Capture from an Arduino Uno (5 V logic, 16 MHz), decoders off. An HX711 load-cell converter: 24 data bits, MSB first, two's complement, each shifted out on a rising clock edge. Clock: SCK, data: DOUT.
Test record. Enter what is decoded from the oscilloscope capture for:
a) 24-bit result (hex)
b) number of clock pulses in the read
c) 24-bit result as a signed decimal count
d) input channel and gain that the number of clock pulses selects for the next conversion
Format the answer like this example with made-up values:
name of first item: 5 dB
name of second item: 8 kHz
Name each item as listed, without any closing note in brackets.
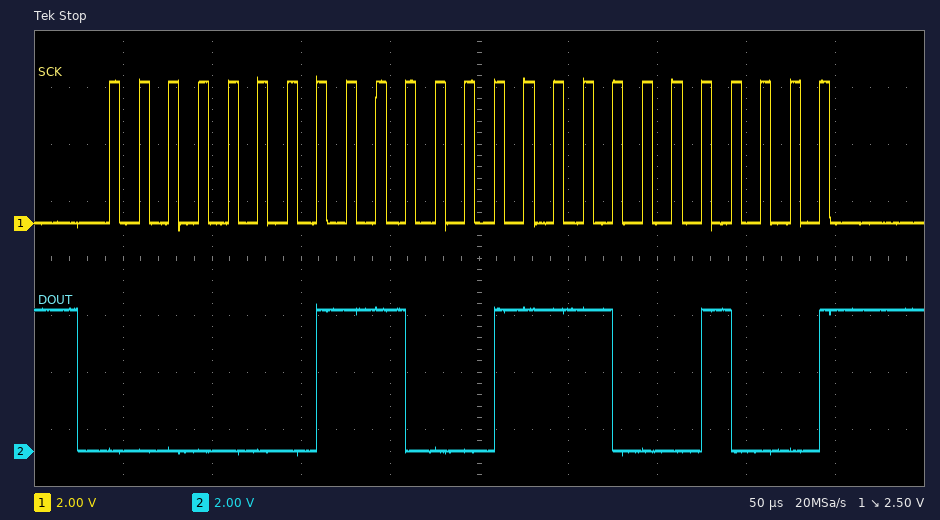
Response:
24-bit result: 0x01C788
number of clock pulses in the read: 25
24-bit result as a signed decimal count: 116616
input channel and gain that the number of clock pulses selects for the next conversion: channel A, gain 128
